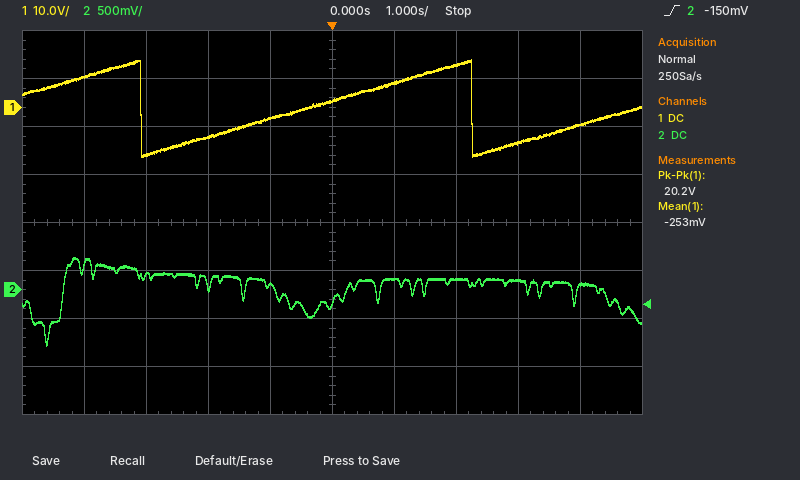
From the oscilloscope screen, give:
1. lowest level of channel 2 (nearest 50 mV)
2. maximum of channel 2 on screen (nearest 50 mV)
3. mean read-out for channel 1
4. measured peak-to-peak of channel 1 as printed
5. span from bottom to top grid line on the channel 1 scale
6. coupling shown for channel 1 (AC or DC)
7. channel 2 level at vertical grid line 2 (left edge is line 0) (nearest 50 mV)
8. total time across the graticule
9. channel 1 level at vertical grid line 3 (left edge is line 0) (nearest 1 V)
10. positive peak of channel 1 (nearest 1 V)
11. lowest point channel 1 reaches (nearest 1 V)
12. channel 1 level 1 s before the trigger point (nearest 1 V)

-600 mV
350 mV
-253 mV
20.2 V
80 V
DC
150 mV
10 s
-6 V
10 V
-10 V
-2 V
